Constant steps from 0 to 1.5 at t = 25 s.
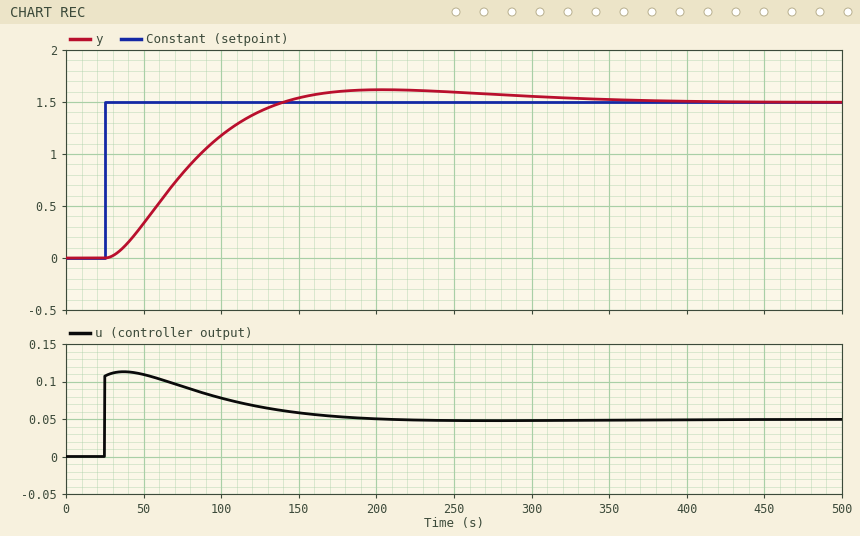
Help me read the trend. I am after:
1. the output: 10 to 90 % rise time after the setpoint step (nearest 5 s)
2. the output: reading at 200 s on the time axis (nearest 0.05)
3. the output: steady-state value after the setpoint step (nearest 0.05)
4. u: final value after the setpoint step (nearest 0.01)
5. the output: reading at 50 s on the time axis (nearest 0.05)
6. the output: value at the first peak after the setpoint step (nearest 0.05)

75 s
1.60
1.50
0.05
0.35
1.60
